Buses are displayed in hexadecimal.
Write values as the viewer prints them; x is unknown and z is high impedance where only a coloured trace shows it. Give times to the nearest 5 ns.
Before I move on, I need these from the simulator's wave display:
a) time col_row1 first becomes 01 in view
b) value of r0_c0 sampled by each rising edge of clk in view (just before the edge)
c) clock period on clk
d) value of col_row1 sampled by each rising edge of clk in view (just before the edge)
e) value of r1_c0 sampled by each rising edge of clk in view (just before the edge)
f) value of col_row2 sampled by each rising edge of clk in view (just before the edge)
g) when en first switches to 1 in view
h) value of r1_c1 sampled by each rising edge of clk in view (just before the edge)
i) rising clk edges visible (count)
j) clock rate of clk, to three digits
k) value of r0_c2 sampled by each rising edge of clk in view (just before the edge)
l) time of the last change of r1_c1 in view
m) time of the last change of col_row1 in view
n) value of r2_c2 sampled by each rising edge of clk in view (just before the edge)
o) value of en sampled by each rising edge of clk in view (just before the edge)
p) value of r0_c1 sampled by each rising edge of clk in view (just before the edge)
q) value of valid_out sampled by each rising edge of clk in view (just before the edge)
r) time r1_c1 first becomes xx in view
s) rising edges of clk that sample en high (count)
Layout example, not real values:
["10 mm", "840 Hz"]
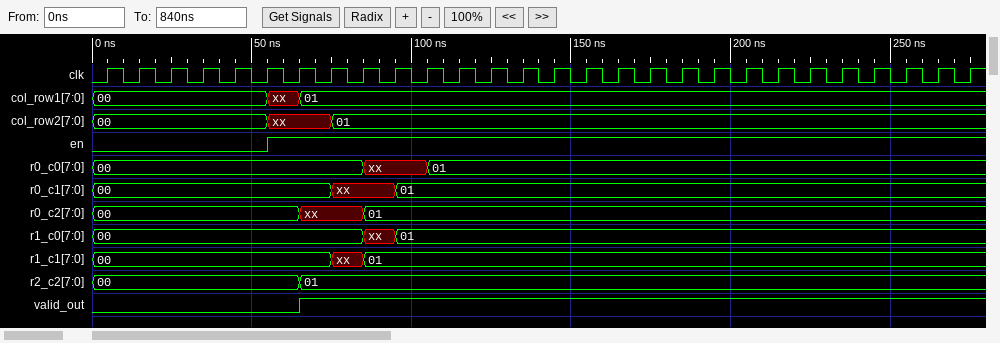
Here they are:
["65 ns", "00, 00, 00, 00, 00, 00, 00, 00, 00, xx, xx, 01, 01, 01, 01, 01, 01, 01, 01, 01, 01, 01, 01, 01, 01, 01, 01, 01", "10 ns", "00, 00, 00, 00, 00, 00, xx, 01, 01, 01, 01, 01, 01, 01, 01, 01, 01, 01, 01, 01, 01, 01, 01, 01, 01, 01, 01, 01", "00, 00, 00, 00, 00, 00, 00, 00, 00, xx, 01, 01, 01, 01, 01, 01, 01, 01, 01, 01, 01, 01, 01, 01, 01, 01, 01, 01", "00, 00, 00, 00, 00, 00, xx, xx, 01, 01, 01, 01, 01, 01, 01, 01, 01, 01, 01, 01, 01, 01, 01, 01, 01, 01, 01, 01", "55 ns", "00, 00, 00, 00, 00, 00, 00, 00, xx, 01, 01, 01, 01, 01, 01, 01, 01, 01, 01, 01, 01, 01, 01, 01, 01, 01, 01, 01", "28", "100 MHz", "00, 00, 00, 00, 00, 00, 00, xx, xx, 01, 01, 01, 01, 01, 01, 01, 01, 01, 01, 01, 01, 01, 01, 01, 01, 01, 01, 01", "85 ns", "65 ns", "00, 00, 00, 00, 00, 00, 00, 01, 01, 01, 01, 01, 01, 01, 01, 01, 01, 01, 01, 01, 01, 01, 01, 01, 01, 01, 01, 01", "0 0 0 0 0 0 1 1 1 1 1 1 1 1 1 1 1 1 1 1 1 1 1 1 1 1 1 1", "00, 00, 00, 00, 00, 00, 00, 00, xx, xx, 01, 01, 01, 01, 01, 01, 01, 01, 01, 01, 01, 01, 01, 01, 01, 01, 01, 01", "0 0 0 0 0 0 0 1 1 1 1 1 1 1 1 1 1 1 1 1 1 1 1 1 1 1 1 1", "75 ns", "22"]
